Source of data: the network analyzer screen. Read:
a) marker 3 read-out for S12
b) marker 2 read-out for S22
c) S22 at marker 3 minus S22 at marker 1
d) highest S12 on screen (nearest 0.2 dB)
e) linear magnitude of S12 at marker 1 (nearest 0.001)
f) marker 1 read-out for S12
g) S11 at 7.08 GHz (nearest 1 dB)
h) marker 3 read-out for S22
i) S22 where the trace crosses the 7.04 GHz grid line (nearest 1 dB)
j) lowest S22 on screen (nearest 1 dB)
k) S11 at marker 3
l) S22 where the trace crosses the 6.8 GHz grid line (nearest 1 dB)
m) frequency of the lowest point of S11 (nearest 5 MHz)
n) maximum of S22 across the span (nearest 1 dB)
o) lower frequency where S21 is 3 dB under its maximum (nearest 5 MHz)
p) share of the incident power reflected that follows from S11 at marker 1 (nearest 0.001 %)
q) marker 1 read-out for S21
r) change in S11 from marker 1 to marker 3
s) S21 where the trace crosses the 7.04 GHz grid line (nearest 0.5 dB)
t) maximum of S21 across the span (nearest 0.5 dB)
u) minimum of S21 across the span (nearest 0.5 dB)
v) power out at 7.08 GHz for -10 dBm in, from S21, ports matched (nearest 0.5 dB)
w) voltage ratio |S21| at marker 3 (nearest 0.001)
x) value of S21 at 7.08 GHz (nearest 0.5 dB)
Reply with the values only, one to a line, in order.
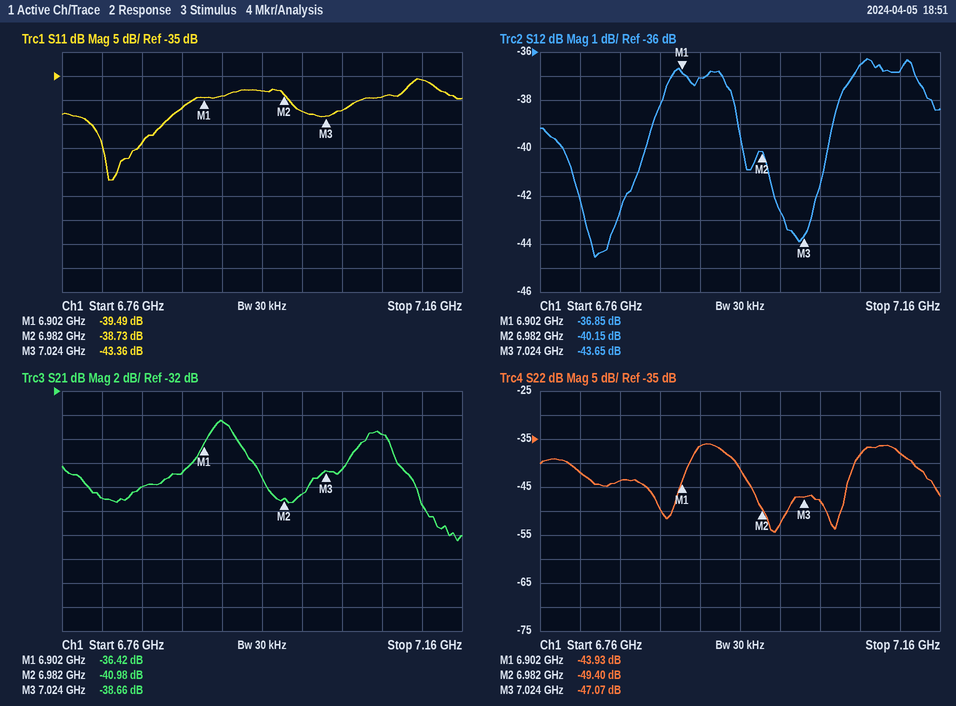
-43.65 dB
-49.40 dB
-3.14 dB
-36.2 dB
0.014
-36.85 dB
-39 dB
-47.07 dB
-48 dB
-54 dB
-43.36 dB
-42 dB
6.805 GHz
-36 dB
6.895 GHz
0.011 %
-36.42 dB
-3.87 dB
-38.5 dB
-34.5 dB
-44.5 dB
-45.5 dBm
0.012
-35.5 dB
